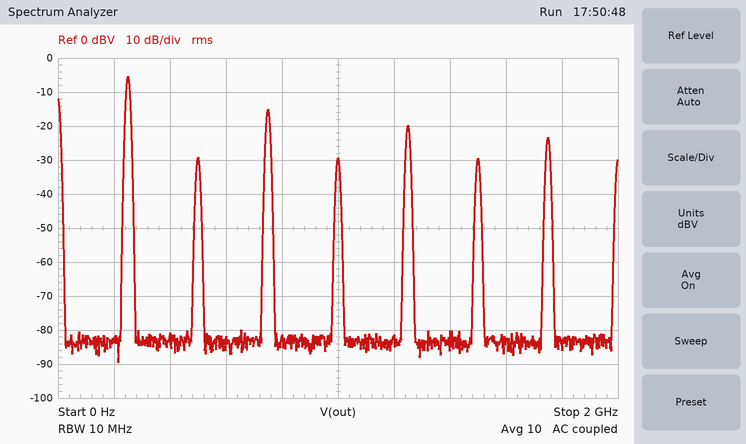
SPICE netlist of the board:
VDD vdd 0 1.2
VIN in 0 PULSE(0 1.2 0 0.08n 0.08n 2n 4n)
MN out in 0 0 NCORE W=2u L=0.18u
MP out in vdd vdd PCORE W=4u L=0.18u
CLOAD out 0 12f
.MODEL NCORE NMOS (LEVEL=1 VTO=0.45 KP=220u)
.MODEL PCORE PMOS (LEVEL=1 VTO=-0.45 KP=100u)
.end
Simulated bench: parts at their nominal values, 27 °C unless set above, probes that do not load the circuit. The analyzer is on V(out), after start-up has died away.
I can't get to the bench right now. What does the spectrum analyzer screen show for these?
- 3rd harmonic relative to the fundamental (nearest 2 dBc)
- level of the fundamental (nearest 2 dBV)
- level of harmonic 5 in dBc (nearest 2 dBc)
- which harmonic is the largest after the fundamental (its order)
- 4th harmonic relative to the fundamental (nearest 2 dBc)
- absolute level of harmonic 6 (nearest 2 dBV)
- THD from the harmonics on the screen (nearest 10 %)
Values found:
-10 dBc
-6 dBV
-14 dBc
3
-24 dBc
-30 dBV
40 %
